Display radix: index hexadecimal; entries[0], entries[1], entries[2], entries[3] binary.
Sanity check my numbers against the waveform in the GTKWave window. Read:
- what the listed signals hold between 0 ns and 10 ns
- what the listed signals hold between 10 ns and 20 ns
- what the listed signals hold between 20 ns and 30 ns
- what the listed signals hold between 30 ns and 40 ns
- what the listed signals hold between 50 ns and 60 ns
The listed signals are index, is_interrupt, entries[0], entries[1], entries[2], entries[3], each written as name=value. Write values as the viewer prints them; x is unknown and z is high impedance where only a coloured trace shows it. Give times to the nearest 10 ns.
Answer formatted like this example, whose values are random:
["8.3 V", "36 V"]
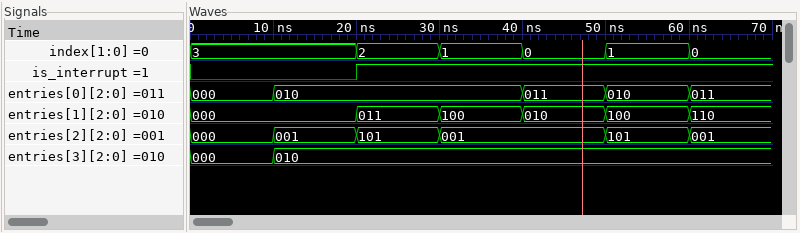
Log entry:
["index=3, is_interrupt=0, entries[0]=000, entries[1]=000, entries[2]=000, entries[3]=000", "index=3, is_interrupt=0, entries[0]=010, entries[1]=000, entries[2]=001, entries[3]=010", "index=2, is_interrupt=1, entries[0]=010, entries[1]=011, entries[2]=101, entries[3]=010", "index=1, is_interrupt=1, entries[0]=010, entries[1]=100, entries[2]=001, entries[3]=010", "index=1, is_interrupt=1, entries[0]=010, entries[1]=100, entries[2]=101, entries[3]=010"]
